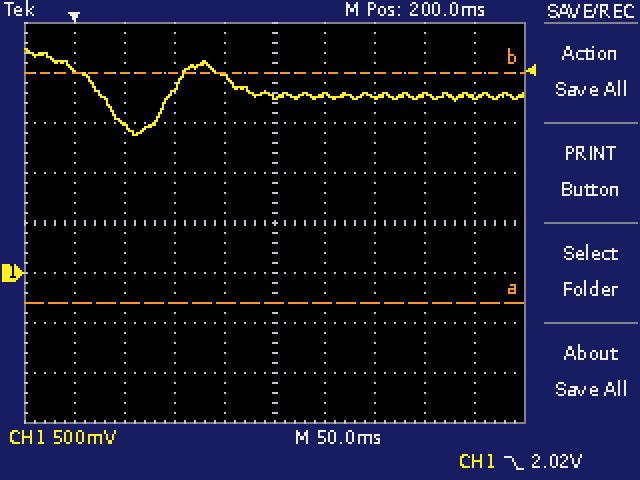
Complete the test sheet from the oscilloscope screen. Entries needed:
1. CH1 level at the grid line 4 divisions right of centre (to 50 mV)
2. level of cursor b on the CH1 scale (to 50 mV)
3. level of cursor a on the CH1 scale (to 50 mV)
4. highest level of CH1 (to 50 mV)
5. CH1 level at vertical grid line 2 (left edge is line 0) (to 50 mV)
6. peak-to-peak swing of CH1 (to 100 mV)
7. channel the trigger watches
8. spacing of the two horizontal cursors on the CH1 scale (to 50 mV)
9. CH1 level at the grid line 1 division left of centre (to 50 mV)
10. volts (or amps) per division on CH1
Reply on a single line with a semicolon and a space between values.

1.75 V; 2.00 V; -300 mV; 2.25 V; 1.50 V; 900 mV; CH1; 2.30 V; 1.95 V; 500 mV
